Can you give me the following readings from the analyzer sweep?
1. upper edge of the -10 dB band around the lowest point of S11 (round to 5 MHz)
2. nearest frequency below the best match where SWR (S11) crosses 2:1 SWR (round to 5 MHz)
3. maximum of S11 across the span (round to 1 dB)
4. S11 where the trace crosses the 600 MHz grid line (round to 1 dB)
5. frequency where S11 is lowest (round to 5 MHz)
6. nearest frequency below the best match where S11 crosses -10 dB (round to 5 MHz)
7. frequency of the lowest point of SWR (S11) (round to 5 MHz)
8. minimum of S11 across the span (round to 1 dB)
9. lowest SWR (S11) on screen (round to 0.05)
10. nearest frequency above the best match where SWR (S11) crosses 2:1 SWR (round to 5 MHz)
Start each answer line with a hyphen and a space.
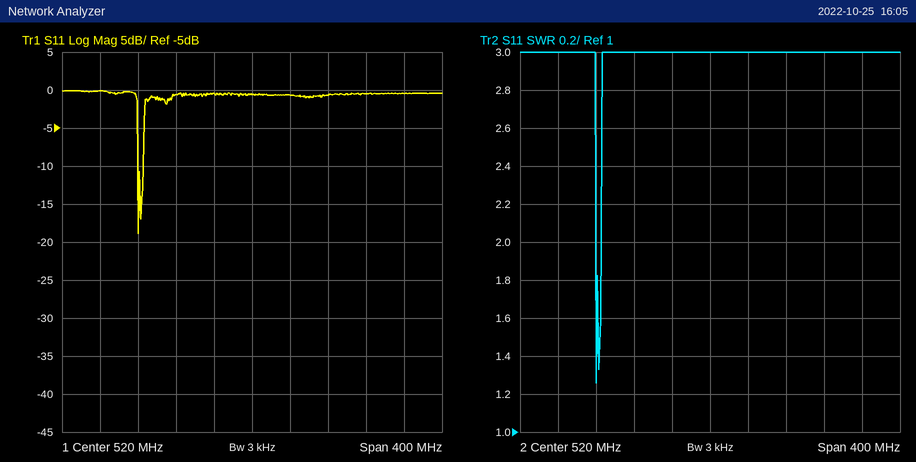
- 405 MHz
- 400 MHz
- 0 dB
- -1 dB
- 400 MHz
- 400 MHz
- 400 MHz
- -19 dB
- 1.25
- 405 MHz
